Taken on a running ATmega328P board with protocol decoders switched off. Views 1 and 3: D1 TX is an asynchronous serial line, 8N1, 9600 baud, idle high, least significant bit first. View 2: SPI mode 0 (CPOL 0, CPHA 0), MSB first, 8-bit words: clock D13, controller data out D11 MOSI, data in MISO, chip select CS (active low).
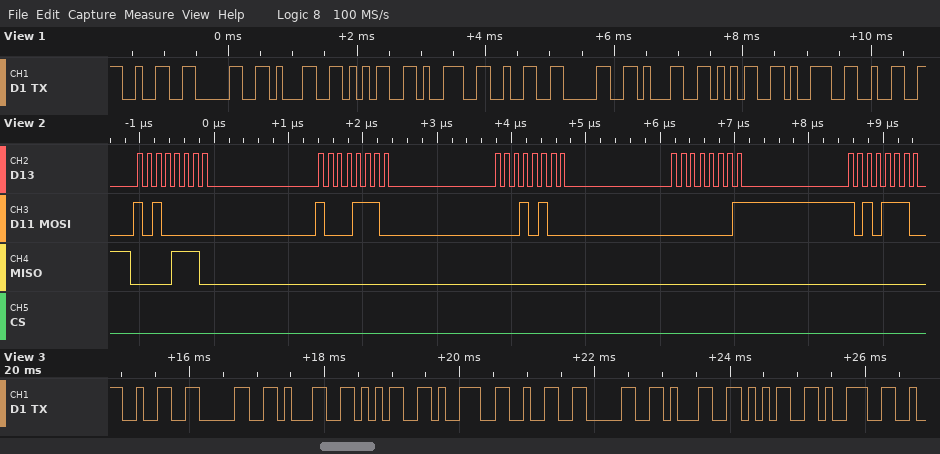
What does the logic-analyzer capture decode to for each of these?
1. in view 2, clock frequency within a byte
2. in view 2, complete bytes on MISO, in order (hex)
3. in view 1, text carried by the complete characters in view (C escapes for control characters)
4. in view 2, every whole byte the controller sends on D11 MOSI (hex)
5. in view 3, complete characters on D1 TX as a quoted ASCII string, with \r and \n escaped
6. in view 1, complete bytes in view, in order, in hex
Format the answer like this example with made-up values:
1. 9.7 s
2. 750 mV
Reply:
1. 8 MHz
2. 0E 00 00 00 00
3. "20159201592"
4. A0 8E 14 01 AE
5. "2015920159"
6. 32 30 31 35 39 32 30 31 35 39 32
